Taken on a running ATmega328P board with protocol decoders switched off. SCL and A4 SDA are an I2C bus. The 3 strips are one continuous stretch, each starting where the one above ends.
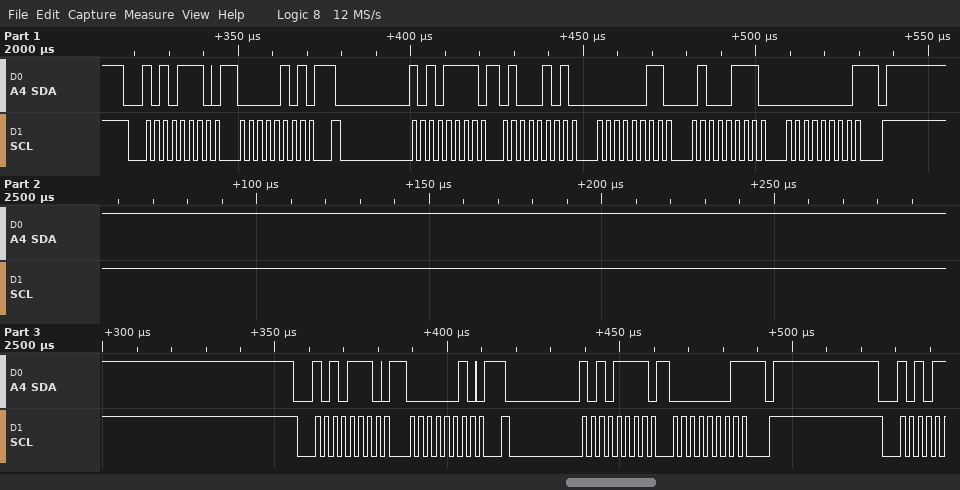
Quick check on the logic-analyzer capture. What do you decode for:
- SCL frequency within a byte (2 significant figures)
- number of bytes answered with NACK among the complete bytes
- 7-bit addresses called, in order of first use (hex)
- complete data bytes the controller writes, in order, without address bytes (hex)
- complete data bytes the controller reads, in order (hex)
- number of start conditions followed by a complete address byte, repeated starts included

400 kHz
2
0x57
05 02
45 03 47 00 01
4
